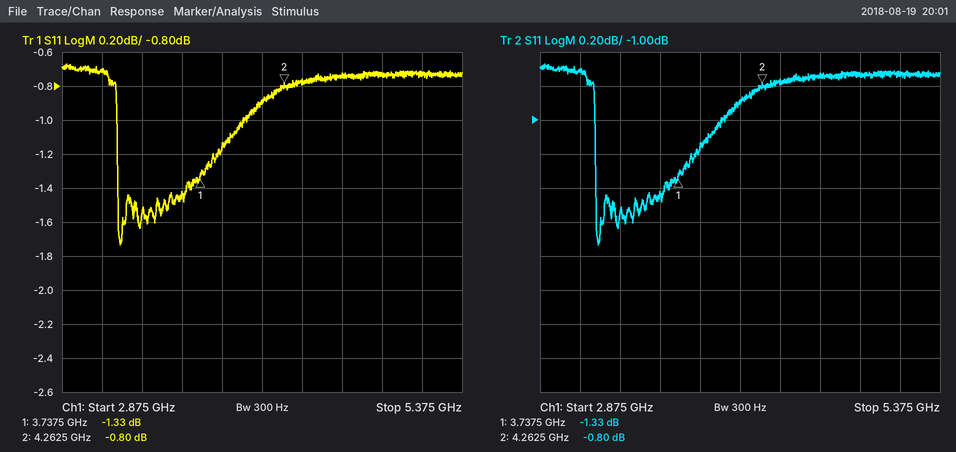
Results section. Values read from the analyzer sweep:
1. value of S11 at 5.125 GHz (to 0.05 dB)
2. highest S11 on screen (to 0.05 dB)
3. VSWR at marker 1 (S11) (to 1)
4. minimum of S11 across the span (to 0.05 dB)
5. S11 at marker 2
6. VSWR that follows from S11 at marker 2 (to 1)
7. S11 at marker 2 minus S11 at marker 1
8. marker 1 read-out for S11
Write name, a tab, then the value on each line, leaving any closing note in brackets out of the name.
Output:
value of S11 at 5.125 GHz	-0.75 dB
highest S11 on screen	-0.65 dB
VSWR at marker 1 (S11)	13
minimum of S11 across the span	-1.75 dB
S11 at marker 2	-0.80 dB
VSWR that follows from S11 at marker 2	22
S11 at marker 2 minus S11 at marker 1	0.53 dB
marker 1 read-out for S11	-1.33 dB
